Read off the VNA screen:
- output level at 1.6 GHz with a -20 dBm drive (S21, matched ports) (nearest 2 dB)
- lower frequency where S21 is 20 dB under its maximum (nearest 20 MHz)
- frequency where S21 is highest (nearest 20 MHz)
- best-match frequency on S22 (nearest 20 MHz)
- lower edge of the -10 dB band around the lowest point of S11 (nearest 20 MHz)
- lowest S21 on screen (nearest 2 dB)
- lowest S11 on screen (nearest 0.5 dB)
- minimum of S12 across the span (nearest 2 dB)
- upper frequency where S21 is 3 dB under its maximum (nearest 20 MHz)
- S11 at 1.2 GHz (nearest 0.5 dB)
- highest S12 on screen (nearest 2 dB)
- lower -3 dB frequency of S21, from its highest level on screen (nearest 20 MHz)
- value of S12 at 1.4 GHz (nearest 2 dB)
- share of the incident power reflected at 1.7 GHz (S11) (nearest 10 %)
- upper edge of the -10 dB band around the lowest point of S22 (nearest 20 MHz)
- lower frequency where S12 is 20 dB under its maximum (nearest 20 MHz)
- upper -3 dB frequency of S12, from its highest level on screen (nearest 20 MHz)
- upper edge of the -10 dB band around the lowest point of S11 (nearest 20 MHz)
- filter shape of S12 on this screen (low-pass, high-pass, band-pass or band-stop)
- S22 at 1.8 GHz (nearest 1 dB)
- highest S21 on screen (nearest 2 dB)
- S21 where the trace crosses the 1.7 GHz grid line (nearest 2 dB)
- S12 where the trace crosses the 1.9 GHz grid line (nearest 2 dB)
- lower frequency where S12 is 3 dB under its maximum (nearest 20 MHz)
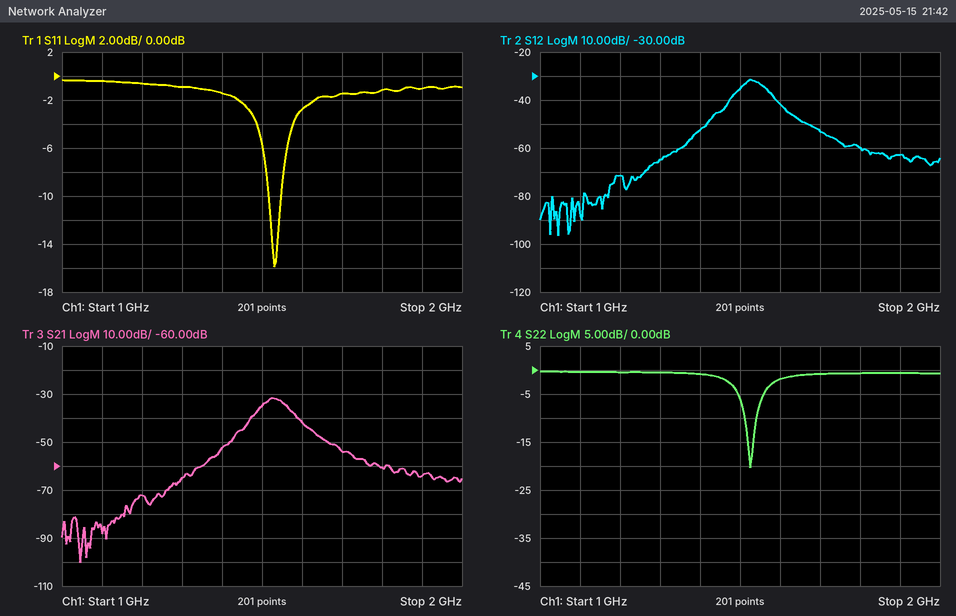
-62 dBm
1.40 GHz
1.52 GHz
1.52 GHz
1.52 GHz
-100 dB
-16.0 dB
-96 dB
1.56 GHz
-0.5 dB
-32 dB
1.50 GHz
-52 dB
70 %
1.54 GHz
1.40 GHz
1.56 GHz
1.54 GHz
band-pass
-1 dB
-32 dB
-54 dB
-62 dB
1.50 GHz
